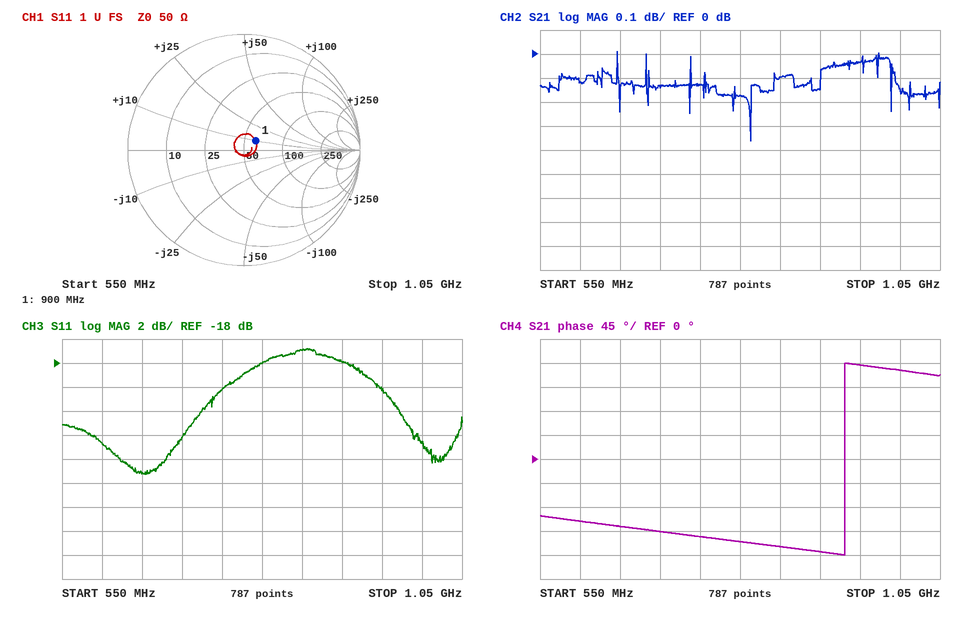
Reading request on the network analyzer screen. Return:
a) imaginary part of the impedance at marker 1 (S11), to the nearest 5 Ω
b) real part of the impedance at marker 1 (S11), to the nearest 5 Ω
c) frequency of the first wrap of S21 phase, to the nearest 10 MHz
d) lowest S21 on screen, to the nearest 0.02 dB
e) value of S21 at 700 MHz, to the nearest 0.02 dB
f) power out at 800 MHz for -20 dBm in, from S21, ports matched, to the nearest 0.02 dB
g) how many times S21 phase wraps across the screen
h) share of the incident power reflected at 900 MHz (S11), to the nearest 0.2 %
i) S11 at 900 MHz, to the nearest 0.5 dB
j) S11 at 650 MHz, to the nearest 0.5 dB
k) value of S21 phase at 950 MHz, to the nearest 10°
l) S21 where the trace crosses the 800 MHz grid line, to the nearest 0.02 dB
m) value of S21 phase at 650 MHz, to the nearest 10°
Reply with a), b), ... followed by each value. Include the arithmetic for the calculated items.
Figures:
a) +10 Ω
b) 60 Ω
c) 930 MHz
d) -0.36 dB
e) -0.14 dB
f) -20 dBm + (-0.18 dB) = -20.18 dBm
g) 1
h) 10^(-18/10) ≈ 1.6 %
i) -18.0 dB
j) -27.0 dB
k) 180°
l) -0.18 dB
m) -130°
